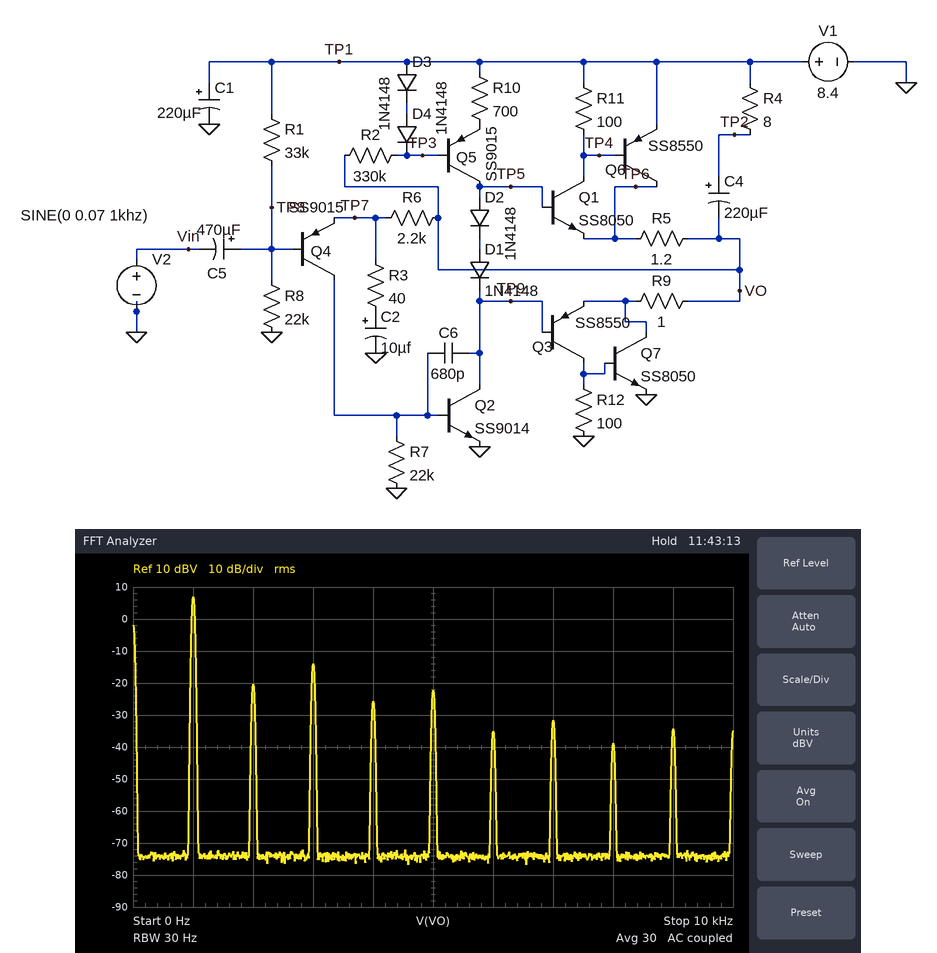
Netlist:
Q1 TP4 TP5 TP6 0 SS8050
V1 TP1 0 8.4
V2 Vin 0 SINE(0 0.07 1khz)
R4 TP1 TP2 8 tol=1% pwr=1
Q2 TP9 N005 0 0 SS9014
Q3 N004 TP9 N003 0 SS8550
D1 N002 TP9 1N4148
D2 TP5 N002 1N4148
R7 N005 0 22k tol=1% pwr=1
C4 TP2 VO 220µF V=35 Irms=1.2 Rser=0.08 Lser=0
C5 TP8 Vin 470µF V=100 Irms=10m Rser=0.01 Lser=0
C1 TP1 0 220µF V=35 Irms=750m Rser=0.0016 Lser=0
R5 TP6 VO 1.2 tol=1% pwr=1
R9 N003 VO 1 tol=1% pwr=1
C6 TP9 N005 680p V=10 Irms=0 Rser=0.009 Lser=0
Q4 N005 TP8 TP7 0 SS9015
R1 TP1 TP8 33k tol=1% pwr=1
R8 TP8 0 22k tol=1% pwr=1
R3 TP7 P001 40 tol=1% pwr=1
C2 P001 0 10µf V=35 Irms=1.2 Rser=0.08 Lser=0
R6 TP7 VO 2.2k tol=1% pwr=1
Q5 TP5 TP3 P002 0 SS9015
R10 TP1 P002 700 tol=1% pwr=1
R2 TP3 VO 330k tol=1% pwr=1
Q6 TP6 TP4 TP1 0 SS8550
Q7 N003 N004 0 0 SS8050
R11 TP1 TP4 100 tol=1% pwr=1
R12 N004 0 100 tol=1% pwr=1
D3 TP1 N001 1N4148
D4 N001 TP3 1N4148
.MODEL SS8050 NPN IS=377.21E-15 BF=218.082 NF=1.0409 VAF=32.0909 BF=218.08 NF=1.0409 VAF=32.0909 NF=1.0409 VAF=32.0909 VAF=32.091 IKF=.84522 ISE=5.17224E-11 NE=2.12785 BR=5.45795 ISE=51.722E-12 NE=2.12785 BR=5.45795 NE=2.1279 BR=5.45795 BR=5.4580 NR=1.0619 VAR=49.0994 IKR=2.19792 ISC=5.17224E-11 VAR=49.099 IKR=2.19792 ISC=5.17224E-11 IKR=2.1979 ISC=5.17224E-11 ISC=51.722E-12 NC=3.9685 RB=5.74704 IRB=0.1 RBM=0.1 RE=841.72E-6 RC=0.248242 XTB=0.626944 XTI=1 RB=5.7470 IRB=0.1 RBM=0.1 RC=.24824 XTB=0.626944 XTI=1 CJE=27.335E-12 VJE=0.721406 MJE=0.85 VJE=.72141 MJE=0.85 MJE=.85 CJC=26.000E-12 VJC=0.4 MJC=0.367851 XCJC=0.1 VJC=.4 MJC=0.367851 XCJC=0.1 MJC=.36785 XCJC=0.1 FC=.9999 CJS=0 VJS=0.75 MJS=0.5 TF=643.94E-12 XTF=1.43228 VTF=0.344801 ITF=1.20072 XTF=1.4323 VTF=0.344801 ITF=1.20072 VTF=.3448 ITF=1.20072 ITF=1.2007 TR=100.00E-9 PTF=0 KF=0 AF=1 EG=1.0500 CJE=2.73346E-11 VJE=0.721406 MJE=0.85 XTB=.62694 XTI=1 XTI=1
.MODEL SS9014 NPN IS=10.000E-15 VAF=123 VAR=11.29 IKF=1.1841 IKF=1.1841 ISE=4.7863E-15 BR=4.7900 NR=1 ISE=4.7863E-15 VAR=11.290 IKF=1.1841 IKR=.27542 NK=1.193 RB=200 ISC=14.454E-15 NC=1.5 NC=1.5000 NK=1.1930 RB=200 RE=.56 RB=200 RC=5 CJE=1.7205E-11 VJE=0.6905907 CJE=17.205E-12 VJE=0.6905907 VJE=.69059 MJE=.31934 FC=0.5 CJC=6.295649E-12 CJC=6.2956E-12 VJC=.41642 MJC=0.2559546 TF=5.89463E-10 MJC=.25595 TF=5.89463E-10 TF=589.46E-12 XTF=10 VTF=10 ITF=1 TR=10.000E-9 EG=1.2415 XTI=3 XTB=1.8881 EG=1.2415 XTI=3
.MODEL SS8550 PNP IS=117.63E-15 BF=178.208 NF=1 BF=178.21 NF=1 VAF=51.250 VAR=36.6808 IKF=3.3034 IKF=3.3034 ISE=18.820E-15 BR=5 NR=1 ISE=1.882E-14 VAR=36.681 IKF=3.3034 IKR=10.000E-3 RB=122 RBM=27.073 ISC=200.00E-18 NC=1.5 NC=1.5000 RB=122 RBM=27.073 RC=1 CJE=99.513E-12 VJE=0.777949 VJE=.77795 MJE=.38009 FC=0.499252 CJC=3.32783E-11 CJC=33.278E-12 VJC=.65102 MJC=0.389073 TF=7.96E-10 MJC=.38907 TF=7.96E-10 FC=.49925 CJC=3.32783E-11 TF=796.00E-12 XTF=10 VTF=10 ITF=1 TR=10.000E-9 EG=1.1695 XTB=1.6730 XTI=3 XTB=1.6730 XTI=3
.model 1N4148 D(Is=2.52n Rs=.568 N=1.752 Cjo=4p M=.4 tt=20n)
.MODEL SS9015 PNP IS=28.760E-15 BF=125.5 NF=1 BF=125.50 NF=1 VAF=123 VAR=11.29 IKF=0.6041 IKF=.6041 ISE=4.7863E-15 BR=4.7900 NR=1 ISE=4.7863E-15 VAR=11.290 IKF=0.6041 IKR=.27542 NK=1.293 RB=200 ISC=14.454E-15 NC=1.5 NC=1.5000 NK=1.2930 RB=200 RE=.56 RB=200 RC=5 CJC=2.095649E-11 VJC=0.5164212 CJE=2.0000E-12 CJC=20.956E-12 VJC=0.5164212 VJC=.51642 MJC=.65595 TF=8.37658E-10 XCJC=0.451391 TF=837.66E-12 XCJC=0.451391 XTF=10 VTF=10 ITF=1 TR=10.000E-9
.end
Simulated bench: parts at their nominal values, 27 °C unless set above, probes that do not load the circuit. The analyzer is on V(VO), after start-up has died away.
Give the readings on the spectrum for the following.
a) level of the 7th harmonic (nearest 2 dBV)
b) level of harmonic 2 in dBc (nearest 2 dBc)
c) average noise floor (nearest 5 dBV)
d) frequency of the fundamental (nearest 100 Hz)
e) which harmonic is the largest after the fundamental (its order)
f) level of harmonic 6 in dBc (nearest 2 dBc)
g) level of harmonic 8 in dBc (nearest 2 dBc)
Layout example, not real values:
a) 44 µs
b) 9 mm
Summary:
a) -32 dBV
b) -28 dBc
c) -75 dBV
d) 1.0 kHz
e) 3
f) -42 dBc
g) -46 dBc
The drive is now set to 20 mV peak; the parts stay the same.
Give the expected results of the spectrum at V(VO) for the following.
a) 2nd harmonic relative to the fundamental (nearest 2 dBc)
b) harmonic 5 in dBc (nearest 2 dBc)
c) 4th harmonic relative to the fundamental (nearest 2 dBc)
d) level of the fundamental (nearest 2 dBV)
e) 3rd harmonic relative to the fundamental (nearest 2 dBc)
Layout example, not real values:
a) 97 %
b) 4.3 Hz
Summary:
a) -34 dBc
b) -34 dBc
c) -46 dBc
d) -2 dBV
e) -30 dBc
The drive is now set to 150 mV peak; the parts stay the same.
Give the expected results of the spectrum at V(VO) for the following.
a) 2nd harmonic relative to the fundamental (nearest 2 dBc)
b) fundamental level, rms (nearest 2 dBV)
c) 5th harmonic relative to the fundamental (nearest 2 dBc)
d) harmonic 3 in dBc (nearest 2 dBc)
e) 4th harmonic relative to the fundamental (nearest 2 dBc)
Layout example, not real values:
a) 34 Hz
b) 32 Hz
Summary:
a) -24 dBc
b) 8 dBV
c) -24 dBc
d) -12 dBc
e) -24 dBc
